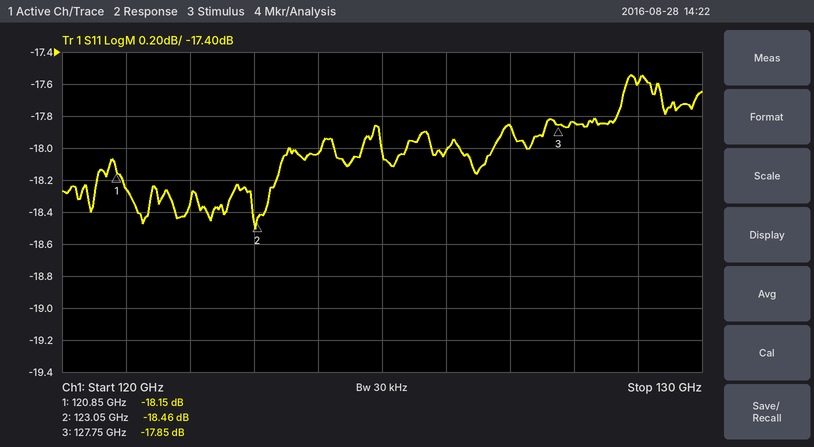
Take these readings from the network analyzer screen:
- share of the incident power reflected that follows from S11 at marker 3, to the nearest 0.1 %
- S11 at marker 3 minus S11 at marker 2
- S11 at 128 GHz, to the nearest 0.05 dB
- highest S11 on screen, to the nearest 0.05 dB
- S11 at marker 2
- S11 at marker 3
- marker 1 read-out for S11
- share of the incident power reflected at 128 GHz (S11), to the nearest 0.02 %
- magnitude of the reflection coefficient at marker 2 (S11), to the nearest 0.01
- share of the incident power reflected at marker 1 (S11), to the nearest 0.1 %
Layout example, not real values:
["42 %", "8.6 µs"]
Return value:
["1.6 %", "0.61 dB", "-17.85 dB", "-17.55 dB", "-18.46 dB", "-17.85 dB", "-18.15 dB", "1.64 %", "0.12", "1.5 %"]
